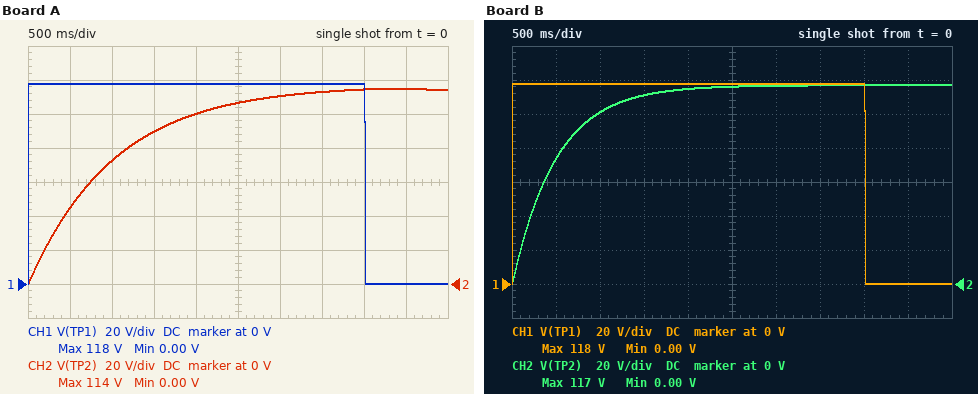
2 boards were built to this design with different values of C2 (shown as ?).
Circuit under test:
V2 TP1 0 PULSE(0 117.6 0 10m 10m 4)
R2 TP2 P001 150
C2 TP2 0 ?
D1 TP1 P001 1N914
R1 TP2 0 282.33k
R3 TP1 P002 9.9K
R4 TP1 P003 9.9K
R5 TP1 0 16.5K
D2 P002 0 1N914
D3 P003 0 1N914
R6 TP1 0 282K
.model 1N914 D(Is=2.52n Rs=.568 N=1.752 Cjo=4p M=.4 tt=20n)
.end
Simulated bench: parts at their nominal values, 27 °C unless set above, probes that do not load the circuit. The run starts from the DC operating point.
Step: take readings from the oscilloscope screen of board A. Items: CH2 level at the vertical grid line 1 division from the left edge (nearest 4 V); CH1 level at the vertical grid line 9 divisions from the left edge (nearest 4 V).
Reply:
44 V
0 V
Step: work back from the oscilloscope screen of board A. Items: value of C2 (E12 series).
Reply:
6.8 mF
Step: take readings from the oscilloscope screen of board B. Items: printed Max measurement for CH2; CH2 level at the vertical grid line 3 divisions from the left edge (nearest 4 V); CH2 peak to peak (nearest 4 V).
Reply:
117 V
112 V
116 V
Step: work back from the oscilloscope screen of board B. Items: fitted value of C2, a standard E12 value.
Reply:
3.3 mF
